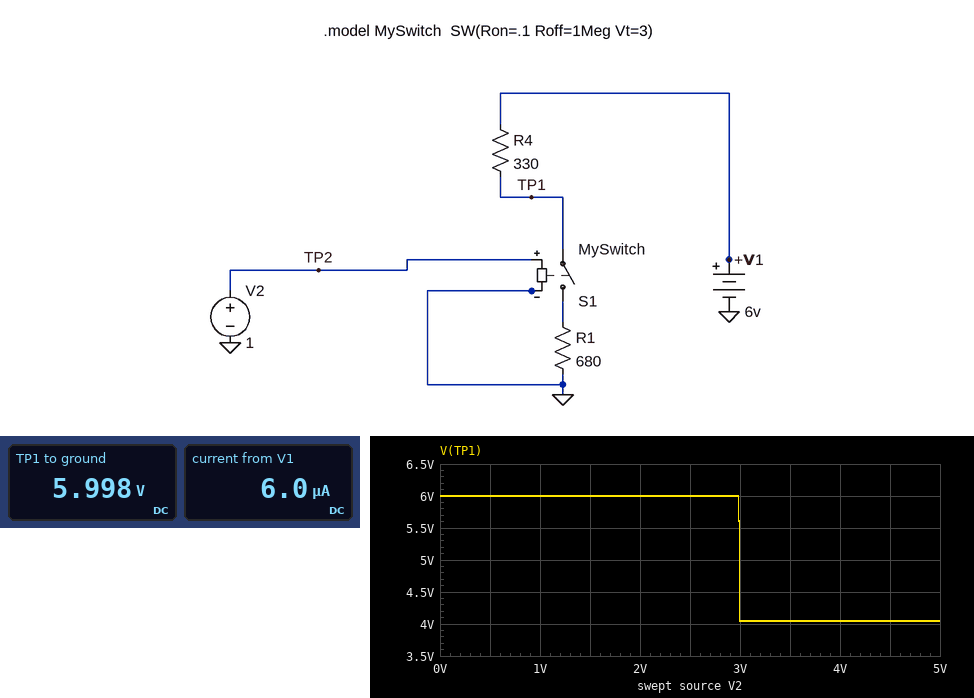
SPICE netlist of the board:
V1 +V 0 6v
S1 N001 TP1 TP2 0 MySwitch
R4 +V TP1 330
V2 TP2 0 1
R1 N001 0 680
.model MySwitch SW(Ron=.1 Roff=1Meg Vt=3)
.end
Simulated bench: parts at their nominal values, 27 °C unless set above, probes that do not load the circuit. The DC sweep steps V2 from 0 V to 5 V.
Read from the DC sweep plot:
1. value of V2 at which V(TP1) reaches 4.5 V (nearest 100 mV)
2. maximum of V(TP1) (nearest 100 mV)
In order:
3.0 V
6.0 V
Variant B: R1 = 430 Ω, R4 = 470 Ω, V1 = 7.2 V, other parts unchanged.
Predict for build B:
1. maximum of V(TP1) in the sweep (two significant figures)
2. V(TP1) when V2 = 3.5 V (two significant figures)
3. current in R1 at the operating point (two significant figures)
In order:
7.2 V
3.4 V
7.2 µA
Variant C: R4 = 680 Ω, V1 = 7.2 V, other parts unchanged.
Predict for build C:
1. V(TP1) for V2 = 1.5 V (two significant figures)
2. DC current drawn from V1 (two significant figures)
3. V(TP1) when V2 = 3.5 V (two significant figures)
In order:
7.2 V
7.2 µA
3.6 V
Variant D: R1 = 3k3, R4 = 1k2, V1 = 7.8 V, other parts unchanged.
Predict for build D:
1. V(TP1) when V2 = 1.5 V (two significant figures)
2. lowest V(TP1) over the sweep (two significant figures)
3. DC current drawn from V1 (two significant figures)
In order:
7.8 V
5.7 V
7.8 µA
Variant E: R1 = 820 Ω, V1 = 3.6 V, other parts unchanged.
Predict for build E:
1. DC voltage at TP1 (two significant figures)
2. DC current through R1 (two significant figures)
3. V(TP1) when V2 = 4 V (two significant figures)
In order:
3.6 V
3.6 µA
2.6 V
